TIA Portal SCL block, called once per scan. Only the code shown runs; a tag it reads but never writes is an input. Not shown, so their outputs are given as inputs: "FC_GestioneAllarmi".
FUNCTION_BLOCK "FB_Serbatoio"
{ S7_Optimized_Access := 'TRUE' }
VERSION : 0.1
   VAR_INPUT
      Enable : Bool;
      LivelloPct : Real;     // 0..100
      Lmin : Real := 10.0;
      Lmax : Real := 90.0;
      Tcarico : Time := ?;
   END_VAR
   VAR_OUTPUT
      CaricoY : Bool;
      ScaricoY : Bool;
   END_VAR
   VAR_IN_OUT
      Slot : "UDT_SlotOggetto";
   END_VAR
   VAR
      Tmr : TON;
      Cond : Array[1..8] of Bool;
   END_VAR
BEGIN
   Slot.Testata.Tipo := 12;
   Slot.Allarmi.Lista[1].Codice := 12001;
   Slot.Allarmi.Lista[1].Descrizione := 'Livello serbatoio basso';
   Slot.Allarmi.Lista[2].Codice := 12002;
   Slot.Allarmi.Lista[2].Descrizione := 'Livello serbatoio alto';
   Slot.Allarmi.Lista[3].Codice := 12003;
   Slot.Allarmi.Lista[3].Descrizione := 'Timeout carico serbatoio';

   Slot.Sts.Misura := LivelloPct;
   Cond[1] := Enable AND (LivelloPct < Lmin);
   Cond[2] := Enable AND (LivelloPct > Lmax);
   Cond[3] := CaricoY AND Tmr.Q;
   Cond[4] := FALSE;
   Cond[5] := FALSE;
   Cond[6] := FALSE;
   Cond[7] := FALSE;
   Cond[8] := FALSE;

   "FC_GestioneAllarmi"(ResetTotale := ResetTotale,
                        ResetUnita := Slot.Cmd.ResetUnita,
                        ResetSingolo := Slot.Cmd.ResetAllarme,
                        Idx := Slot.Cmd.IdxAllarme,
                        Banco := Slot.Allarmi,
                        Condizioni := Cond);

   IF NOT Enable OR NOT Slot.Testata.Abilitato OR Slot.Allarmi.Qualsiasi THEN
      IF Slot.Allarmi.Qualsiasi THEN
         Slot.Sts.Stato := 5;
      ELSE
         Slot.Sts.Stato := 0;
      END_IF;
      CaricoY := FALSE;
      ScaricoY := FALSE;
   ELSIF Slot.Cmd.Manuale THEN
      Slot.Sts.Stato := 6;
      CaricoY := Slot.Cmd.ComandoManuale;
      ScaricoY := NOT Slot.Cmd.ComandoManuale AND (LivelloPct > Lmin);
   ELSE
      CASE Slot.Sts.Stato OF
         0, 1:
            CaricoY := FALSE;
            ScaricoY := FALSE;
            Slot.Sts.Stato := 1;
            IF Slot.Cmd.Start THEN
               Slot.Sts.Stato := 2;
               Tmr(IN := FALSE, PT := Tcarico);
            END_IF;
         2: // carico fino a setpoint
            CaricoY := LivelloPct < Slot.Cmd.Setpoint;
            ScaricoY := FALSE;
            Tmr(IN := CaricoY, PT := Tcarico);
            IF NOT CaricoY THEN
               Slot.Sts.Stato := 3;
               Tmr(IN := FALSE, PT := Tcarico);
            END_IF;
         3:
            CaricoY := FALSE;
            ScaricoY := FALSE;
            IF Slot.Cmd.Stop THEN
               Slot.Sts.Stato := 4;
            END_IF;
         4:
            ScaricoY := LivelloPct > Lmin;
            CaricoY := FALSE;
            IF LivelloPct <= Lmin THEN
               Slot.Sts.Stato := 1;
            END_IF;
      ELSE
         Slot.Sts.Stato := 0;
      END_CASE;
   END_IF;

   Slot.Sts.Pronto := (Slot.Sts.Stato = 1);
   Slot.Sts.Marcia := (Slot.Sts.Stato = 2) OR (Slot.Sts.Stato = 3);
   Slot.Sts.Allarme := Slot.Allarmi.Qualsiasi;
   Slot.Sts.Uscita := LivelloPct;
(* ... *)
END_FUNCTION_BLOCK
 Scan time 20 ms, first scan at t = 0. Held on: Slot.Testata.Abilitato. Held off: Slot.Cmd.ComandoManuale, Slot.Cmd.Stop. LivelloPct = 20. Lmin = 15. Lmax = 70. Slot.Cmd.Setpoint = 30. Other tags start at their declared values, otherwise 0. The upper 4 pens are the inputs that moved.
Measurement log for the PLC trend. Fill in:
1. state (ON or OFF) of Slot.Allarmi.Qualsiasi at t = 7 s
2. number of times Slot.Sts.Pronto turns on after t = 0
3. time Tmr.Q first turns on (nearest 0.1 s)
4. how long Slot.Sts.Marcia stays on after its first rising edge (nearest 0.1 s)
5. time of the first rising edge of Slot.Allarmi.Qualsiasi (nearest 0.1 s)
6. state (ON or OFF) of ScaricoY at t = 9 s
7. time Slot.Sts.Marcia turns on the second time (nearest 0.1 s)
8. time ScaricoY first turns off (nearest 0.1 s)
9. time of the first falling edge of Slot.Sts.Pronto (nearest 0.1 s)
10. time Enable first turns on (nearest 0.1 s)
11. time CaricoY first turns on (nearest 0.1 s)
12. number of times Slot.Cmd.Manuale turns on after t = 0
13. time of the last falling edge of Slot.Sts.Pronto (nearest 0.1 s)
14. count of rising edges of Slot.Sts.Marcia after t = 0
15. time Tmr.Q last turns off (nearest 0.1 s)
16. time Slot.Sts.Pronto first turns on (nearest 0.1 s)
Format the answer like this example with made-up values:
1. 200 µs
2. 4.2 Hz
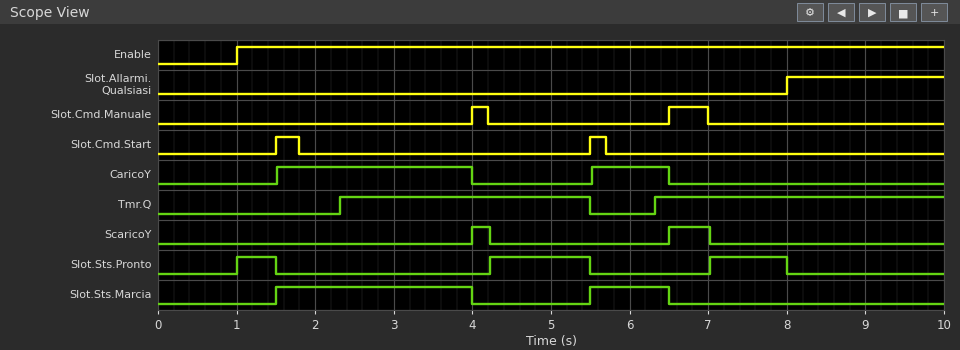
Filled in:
1. OFF
2. 3
3. 2.3 s
4. 2.5 s
5. 8.0 s
6. OFF
7. 5.5 s
8. 4.2 s
9. 1.5 s
10. 1.0 s
11. 1.5 s
12. 2
13. 8.0 s
14. 2
15. 5.5 s
16. 1.0 s
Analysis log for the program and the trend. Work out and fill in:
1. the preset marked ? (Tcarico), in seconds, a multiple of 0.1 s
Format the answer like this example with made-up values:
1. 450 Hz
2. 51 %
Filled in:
1. 0.8 s
